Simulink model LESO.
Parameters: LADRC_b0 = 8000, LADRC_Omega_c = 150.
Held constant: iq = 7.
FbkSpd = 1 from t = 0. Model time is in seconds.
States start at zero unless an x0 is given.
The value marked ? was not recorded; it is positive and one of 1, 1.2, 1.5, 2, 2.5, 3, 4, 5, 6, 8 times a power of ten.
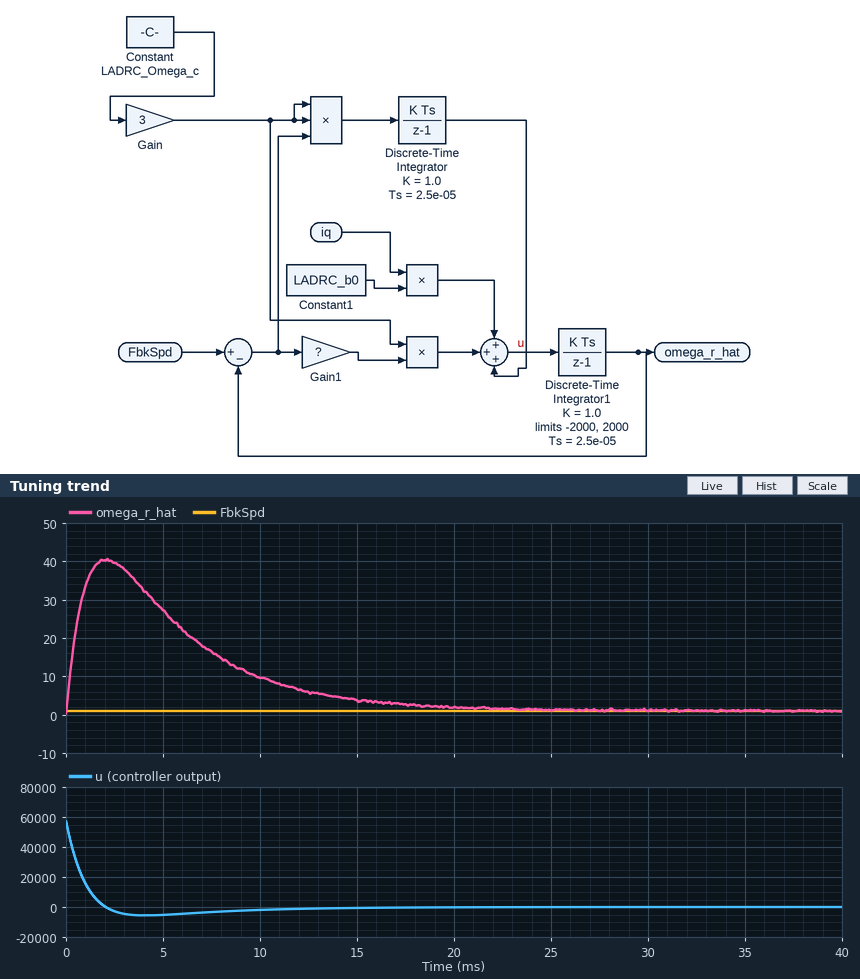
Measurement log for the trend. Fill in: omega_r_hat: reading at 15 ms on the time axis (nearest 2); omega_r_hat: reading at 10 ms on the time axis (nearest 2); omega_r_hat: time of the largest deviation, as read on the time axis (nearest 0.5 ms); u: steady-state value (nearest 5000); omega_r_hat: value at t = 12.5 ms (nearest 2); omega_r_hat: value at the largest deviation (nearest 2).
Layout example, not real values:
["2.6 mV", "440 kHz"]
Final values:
["4", "10", "2.0 ms", "0", "6", "40"]
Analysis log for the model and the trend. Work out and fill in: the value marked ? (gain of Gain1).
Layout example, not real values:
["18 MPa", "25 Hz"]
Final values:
["2.5"]
